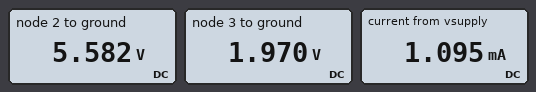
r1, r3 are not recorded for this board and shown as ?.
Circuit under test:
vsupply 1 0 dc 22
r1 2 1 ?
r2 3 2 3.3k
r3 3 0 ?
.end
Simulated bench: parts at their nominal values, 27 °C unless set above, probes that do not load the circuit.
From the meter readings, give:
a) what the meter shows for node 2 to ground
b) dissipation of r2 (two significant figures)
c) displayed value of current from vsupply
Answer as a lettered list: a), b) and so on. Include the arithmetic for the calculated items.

a) 5.582 V
b) (5.582 V - 1.97 V)^2 / 3.3 kΩ = 4.0 mW
c) 1.095 mA
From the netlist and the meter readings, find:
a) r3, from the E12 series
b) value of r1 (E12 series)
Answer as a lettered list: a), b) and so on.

a) 1.8 kΩ
b) 15 kΩ
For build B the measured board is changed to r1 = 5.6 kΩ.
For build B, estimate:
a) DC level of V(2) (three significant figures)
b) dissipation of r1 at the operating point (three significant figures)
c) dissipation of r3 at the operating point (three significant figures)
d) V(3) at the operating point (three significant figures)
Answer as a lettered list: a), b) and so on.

a) 10.5 V
b) 23.7 mW
c) 7.61 mW
d) 3.70 V
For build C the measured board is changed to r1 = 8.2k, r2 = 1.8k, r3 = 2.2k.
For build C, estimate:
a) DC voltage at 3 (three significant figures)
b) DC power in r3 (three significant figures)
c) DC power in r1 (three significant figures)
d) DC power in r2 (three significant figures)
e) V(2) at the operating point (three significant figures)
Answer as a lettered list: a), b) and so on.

a) 3.97 V
b) 7.15 mW
c) 26.7 mW
d) 5.85 mW
e) 7.21 V
